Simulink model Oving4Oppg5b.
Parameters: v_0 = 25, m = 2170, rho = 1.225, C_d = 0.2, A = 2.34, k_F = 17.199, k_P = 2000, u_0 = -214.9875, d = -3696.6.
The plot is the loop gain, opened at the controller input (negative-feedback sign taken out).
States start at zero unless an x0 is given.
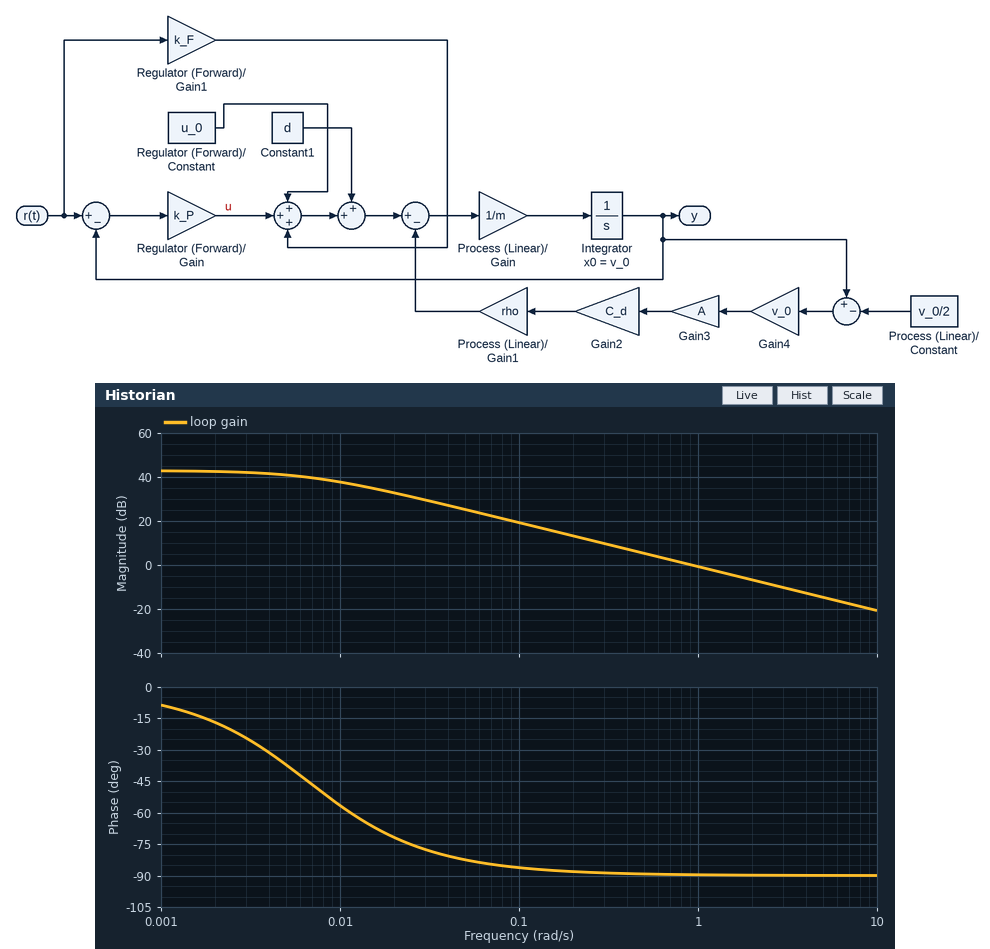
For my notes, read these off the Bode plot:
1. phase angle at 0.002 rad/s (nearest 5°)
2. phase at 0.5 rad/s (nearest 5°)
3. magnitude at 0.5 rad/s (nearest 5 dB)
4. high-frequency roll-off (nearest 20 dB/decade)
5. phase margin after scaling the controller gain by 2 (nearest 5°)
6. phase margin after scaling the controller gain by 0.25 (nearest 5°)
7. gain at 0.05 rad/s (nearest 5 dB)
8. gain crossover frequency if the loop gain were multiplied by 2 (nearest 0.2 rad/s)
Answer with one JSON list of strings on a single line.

["-15°", "-90°", "5 dB", "-20 dB/decade", "90°", "90°", "25 dB", "1.8 rad/s"]
